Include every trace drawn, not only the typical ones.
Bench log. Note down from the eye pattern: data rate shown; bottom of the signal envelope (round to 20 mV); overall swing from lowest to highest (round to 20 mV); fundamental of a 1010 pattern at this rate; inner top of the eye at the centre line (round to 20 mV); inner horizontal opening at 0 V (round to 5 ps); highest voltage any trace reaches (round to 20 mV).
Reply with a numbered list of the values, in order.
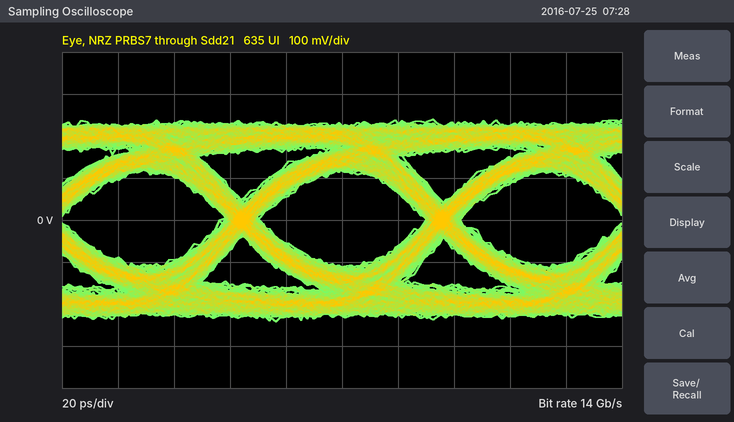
1. 14 Gb/s
2. -240 mV
3. 480 mV
4. 7 GHz
5. 120 mV
6. 60 ps
7. 240 mV
